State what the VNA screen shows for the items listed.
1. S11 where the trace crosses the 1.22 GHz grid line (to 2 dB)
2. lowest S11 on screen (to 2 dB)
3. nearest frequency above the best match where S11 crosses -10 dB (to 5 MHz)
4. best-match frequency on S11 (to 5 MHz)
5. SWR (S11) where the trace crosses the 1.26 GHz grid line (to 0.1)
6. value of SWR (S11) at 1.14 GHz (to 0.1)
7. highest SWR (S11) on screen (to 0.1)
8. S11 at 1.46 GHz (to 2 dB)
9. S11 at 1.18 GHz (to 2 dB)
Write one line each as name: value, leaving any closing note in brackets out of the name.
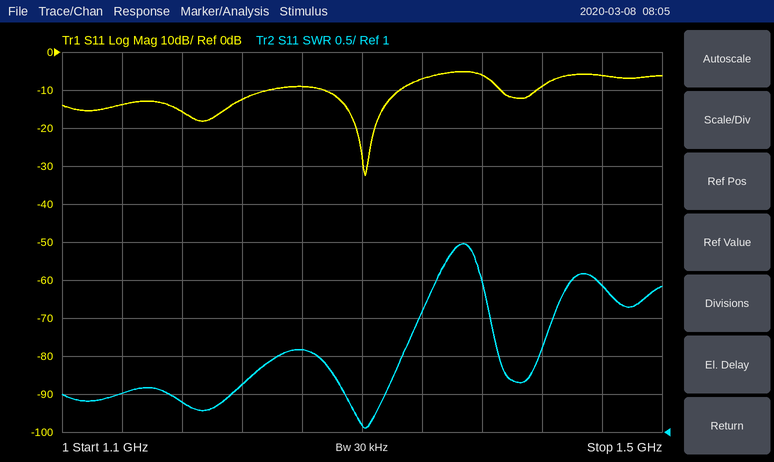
S11 where the trace crosses the 1.22 GHz grid line: -12 dB
lowest S11 on screen: -32 dB
nearest frequency above the best match where S11 crosses -10 dB: 1.325 GHz
best-match frequency on S11: 1.300 GHz
SWR (S11) where the trace crosses the 1.26 GHz grid line: 2.1
value of SWR (S11) at 1.14 GHz: 1.5
highest SWR (S11) on screen: 3.5
S11 at 1.46 GHz: -6 dB
S11 at 1.18 GHz: -16 dB
